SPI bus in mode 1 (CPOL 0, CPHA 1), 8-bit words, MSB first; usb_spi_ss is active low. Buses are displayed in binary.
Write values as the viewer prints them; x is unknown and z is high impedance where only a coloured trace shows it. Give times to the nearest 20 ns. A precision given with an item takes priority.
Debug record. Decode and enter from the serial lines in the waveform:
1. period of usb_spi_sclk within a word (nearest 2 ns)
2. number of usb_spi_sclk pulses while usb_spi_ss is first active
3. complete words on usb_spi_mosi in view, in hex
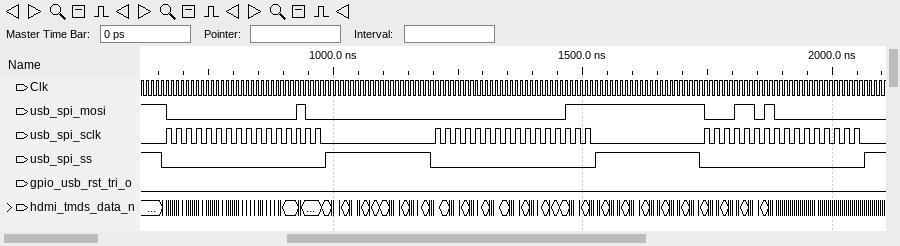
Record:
20 ns
16
00, 04, 00, 07, 1A, 00
